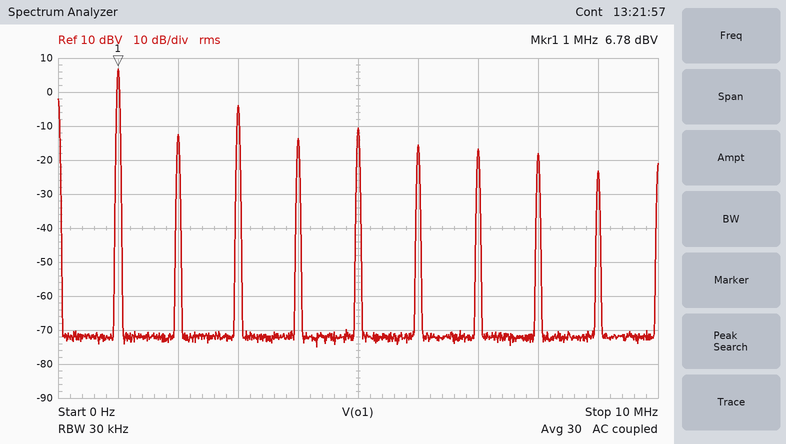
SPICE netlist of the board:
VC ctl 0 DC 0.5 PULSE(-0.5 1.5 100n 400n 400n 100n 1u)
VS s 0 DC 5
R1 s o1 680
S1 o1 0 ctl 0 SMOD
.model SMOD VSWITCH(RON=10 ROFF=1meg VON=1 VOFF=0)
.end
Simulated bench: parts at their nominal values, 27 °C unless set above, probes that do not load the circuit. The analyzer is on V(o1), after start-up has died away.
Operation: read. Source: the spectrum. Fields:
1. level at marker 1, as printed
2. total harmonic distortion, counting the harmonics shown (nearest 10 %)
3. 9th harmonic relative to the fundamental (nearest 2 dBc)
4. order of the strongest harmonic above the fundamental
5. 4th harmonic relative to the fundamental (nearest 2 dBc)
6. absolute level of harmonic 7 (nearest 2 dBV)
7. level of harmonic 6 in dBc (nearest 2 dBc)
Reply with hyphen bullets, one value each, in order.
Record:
- 6.78 dBV
- 40 %
- -30 dBc
- 3
- -20 dBc
- -16 dBV
- -22 dBc
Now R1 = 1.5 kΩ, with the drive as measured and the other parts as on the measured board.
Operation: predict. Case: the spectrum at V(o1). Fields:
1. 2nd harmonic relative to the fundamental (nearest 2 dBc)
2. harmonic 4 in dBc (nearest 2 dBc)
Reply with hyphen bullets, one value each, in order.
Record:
- -26 dBc
- -26 dBc
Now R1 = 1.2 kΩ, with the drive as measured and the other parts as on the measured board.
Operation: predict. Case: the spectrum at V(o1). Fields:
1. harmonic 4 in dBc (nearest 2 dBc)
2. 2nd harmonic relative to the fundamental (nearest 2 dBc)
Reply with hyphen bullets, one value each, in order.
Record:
- -24 dBc
- -24 dBc
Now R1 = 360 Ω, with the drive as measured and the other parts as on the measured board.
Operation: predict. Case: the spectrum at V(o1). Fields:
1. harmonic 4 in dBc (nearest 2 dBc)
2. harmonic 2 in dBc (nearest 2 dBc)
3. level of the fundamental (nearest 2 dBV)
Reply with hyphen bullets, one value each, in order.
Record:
- -18 dBc
- -16 dBc
- 6 dBV
